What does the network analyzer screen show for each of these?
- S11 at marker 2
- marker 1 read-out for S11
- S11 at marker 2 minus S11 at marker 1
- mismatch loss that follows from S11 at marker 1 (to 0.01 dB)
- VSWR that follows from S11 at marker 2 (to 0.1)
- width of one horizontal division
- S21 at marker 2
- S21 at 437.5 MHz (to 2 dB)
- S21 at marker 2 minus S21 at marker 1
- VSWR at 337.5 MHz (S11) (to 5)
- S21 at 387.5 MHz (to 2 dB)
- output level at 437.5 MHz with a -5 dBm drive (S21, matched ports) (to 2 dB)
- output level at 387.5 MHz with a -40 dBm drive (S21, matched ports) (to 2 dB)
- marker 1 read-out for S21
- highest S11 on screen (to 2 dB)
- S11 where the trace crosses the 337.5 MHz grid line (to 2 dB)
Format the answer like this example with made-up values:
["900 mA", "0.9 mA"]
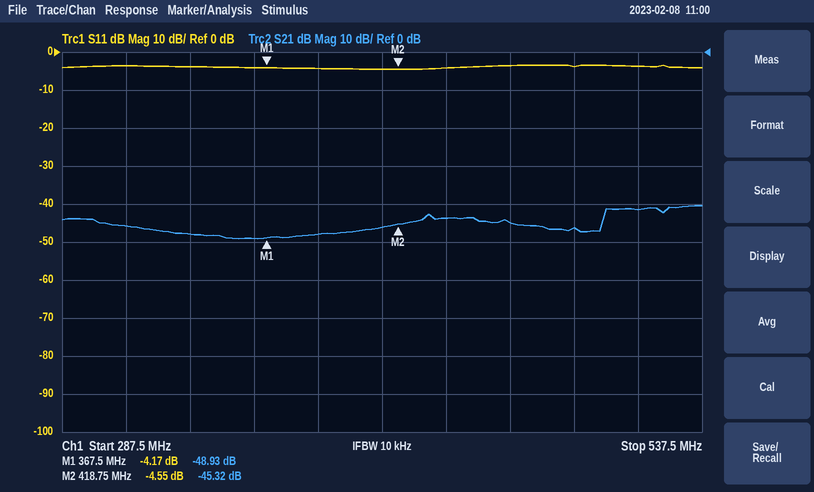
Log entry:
["-4.55 dB", "-4.17 dB", "-0.38 dB", "2.10 dB", "3.9", "25 MHz", "-45.32 dB", "-44 dB", "3.61 dB", "5", "-48 dB", "-48 dBm", "-88 dBm", "-48.93 dB", "-4 dB", "-4 dB"]
